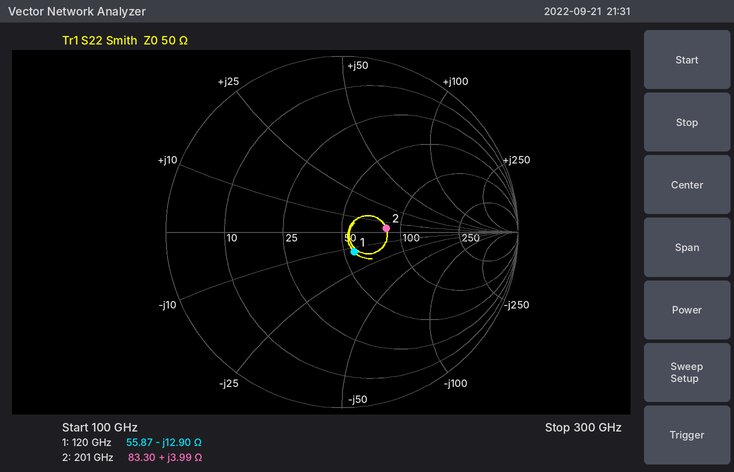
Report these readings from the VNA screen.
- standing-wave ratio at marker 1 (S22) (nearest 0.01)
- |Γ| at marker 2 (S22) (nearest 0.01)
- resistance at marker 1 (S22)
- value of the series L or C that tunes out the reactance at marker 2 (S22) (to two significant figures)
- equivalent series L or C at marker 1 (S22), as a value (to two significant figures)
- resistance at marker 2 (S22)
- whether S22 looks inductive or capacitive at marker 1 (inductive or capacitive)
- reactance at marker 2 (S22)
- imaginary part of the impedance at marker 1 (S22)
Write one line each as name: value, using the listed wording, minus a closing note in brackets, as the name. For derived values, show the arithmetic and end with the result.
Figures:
standing-wave ratio at marker 1 (S22): 1.31
|Γ| at marker 2 (S22): 0.25
resistance at marker 1: 55.87 Ω
value of the series L or C that tunes out the reactance at marker 2 (S22): C = 1/(2π × 201 GHz × 3.99 Ω) ≈ 198 fF, so 200 fF to two significant figures
equivalent series L or C at marker 1 (S22), as a value: C = 1/(2π × 120 GHz × 12.9 Ω) ≈ 103 fF, so 100 fF to two significant figures
resistance at marker 2: 83.30 Ω
whether S22 looks inductive or capacitive at marker 1: capacitive
reactance at marker 2: +3.99 Ω
imaginary part of the impedance at marker 1: -12.90 Ω
